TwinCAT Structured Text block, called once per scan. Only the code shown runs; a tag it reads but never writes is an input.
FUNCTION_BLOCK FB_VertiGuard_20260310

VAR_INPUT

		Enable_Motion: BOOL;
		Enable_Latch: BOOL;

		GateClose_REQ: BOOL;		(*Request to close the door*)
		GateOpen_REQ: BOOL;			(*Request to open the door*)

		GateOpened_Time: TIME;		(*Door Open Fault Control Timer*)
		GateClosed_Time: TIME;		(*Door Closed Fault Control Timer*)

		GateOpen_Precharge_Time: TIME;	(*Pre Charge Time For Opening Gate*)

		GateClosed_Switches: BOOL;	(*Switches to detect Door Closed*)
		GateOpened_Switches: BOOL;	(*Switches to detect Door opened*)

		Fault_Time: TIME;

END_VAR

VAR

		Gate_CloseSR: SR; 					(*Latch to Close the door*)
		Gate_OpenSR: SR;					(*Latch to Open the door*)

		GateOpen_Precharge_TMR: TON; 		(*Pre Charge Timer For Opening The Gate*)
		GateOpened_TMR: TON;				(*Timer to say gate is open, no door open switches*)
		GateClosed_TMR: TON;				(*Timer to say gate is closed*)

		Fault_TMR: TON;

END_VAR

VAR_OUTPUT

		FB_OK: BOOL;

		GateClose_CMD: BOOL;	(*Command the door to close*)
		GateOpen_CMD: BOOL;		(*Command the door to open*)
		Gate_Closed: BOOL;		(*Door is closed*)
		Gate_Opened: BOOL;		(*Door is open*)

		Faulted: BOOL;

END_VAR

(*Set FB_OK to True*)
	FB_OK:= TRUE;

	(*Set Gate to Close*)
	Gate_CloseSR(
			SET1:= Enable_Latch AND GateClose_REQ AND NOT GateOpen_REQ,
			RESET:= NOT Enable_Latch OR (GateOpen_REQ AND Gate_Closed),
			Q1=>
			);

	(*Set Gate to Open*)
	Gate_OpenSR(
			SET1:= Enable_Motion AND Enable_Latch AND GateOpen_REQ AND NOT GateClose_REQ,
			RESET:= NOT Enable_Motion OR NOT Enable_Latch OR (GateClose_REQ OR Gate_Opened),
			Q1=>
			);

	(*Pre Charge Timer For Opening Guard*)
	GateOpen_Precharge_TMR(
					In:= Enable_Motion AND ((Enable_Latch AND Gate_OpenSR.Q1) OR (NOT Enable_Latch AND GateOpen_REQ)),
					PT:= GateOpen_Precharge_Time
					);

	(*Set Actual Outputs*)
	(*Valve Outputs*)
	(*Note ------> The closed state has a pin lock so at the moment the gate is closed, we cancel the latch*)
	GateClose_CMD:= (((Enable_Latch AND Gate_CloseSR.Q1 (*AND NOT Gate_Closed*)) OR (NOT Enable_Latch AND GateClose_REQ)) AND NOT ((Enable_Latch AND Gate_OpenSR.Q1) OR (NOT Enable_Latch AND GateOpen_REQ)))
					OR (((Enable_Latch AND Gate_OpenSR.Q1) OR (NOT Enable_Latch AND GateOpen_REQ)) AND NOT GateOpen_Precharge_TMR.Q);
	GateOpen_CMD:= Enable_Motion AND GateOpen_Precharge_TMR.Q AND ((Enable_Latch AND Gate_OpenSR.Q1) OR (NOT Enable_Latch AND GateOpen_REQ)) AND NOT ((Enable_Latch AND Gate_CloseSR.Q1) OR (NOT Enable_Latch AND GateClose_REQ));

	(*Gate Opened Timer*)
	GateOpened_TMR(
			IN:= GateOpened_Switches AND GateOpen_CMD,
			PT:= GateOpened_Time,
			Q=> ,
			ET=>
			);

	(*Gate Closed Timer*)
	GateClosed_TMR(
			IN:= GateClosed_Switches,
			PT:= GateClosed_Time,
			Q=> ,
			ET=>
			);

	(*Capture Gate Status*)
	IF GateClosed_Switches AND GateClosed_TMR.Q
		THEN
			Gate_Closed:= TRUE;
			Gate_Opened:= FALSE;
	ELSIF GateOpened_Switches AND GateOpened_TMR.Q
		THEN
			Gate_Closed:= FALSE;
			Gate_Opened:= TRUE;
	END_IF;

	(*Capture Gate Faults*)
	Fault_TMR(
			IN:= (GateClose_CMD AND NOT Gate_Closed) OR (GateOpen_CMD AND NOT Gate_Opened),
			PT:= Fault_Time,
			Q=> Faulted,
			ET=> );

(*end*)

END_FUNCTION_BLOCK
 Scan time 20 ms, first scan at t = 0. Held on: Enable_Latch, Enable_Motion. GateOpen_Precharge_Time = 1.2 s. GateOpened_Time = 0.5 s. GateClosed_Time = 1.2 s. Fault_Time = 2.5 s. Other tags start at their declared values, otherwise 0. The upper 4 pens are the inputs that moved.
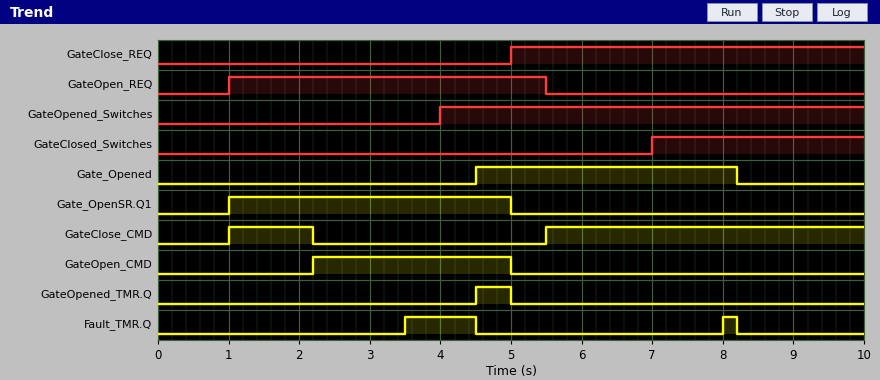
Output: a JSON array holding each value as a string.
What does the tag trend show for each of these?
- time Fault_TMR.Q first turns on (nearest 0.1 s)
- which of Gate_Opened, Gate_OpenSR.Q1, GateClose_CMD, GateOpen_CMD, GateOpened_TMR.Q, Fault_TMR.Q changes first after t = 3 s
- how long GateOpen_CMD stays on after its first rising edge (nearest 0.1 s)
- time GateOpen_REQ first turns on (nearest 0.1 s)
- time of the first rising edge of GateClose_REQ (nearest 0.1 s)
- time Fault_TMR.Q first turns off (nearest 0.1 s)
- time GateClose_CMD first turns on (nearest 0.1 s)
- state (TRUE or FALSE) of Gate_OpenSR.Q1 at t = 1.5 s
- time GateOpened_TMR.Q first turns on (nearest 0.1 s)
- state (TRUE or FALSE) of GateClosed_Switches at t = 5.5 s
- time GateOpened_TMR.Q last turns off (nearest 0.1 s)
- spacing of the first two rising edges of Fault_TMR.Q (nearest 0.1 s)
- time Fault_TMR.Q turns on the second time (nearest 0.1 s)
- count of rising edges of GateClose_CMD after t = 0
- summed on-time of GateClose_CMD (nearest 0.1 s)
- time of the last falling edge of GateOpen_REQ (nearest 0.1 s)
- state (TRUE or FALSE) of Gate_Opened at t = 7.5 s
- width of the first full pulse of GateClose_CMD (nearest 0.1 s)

["3.5 s", "Fault_TMR.Q", "2.8 s", "1.0 s", "5.0 s", "4.5 s", "1.0 s", "TRUE", "4.5 s", "FALSE", "5.0 s", "4.5 s", "8.0 s", "2", "5.7 s", "5.5 s", "TRUE", "1.2 s"]
